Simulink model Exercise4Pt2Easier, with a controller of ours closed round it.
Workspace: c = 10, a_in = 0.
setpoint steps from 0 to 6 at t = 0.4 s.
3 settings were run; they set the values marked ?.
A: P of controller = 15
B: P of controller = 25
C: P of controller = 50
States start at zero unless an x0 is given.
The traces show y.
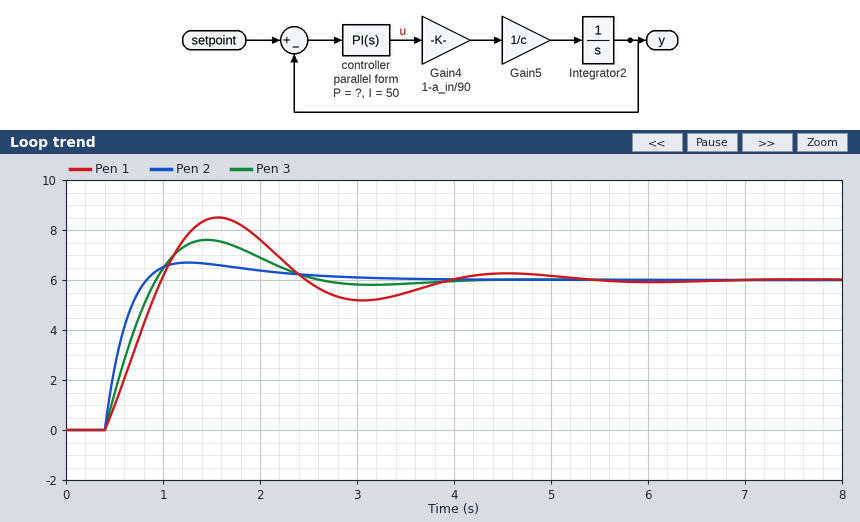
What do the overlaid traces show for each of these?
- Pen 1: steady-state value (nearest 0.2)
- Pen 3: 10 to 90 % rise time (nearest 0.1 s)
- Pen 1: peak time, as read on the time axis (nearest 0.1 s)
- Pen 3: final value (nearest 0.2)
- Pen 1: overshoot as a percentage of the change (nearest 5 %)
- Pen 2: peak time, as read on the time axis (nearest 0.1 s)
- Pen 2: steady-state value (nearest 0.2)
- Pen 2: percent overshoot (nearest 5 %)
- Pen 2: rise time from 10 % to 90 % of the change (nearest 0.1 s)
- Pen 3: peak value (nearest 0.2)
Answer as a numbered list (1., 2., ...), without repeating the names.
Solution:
1. 6.0
2. 0.4 s
3. 1.6 s
4. 6.0
5. 40 %
6. 1.3 s
7. 6.0
8. 10 %
9. 0.3 s
10. 7.6
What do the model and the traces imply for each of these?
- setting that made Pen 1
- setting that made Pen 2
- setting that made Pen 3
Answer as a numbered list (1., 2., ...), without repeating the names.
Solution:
1. A
2. C
3. B
